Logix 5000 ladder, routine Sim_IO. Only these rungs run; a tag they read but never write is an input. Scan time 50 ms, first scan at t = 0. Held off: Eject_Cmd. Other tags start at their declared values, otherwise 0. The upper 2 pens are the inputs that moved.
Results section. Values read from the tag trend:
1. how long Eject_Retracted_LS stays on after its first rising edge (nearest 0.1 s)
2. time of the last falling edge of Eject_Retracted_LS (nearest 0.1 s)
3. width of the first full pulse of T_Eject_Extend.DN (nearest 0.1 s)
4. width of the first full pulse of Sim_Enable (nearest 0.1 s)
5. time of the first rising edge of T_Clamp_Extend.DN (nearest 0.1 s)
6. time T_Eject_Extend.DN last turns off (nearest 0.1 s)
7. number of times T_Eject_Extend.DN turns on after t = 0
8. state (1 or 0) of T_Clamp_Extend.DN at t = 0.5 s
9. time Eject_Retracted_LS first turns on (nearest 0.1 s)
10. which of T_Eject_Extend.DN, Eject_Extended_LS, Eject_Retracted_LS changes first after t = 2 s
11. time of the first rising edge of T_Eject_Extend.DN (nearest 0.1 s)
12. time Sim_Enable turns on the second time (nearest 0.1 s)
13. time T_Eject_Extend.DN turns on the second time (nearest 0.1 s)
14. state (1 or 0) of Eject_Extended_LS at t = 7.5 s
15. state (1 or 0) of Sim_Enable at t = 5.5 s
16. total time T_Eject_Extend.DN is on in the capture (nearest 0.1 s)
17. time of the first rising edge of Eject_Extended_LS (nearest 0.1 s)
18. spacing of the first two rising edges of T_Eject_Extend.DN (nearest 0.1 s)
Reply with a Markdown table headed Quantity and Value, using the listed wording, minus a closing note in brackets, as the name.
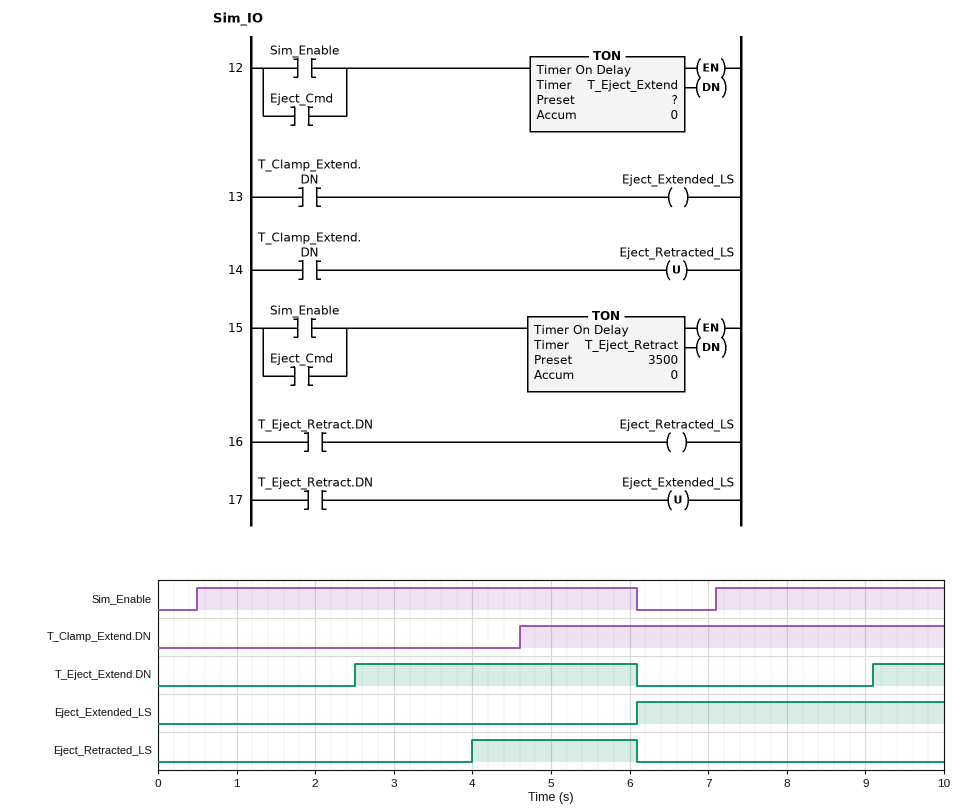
| Quantity | Value |
|---|---|
| how long Eject_Retracted_LS stays on after its first rising edge | 2.1 s |
| time of the last falling edge of Eject_Retracted_LS | 6.1 s |
| width of the first full pulse of T_Eject_Extend.DN | 3.6 s |
| width of the first full pulse of Sim_Enable | 5.6 s |
| time of the first rising edge of T_Clamp_Extend.DN | 4.6 s |
| time T_Eject_Extend.DN last turns off | 6.1 s |
| number of times T_Eject_Extend.DN turns on after t = 0 | 2 |
| state (1 or 0) of T_Clamp_Extend.DN at t = 0.5 s | 0 |
| time Eject_Retracted_LS first turns on | 4.0 s |
| which of T_Eject_Extend.DN, Eject_Extended_LS, Eject_Retracted_LS changes first after t = 2 s | T_Eject_Extend.DN |
| time of the first rising edge of T_Eject_Extend.DN | 2.5 s |
| time Sim_Enable turns on the second time | 7.1 s |
| time T_Eject_Extend.DN turns on the second time | 9.1 s |
| state (1 or 0) of Eject_Extended_LS at t = 7.5 s | 1 |
| state (1 or 0) of Sim_Enable at t = 5.5 s | 1 |
| total time T_Eject_Extend.DN is on in the capture | 4.5 s |
| time of the first rising edge of Eject_Extended_LS | 6.1 s |
| spacing of the first two rising edges of T_Eject_Extend.DN | 6.6 s |
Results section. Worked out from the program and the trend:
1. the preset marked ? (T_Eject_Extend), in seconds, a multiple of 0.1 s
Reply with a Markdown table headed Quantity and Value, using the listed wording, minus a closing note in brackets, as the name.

| Quantity | Value |
|---|---|
| the preset marked ? (T_Eject_Extend), in seconds, a multiple of 0.1 s | 2.0 s |
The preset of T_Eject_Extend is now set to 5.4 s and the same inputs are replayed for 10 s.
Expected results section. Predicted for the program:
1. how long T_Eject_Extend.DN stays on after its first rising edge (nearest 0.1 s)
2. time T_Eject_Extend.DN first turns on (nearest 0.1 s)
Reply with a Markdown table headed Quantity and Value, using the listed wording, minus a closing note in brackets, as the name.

| Quantity | Value |
|---|---|
| how long T_Eject_Extend.DN stays on after its first rising edge | 0.2 s |
| time T_Eject_Extend.DN first turns on | 5.9 s |
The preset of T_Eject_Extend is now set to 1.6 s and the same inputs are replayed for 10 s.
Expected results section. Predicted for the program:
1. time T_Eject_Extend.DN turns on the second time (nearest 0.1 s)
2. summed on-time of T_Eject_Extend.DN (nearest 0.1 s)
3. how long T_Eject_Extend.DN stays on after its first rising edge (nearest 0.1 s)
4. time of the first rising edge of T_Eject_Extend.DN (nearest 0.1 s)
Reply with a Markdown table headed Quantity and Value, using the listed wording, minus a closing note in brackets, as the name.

| Quantity | Value |
|---|---|
| time T_Eject_Extend.DN turns on the second time | 8.7 s |
| summed on-time of T_Eject_Extend.DN | 5.3 s |
| how long T_Eject_Extend.DN stays on after its first rising edge | 4.0 s |
| time of the first rising edge of T_Eject_Extend.DN | 2.1 s |
